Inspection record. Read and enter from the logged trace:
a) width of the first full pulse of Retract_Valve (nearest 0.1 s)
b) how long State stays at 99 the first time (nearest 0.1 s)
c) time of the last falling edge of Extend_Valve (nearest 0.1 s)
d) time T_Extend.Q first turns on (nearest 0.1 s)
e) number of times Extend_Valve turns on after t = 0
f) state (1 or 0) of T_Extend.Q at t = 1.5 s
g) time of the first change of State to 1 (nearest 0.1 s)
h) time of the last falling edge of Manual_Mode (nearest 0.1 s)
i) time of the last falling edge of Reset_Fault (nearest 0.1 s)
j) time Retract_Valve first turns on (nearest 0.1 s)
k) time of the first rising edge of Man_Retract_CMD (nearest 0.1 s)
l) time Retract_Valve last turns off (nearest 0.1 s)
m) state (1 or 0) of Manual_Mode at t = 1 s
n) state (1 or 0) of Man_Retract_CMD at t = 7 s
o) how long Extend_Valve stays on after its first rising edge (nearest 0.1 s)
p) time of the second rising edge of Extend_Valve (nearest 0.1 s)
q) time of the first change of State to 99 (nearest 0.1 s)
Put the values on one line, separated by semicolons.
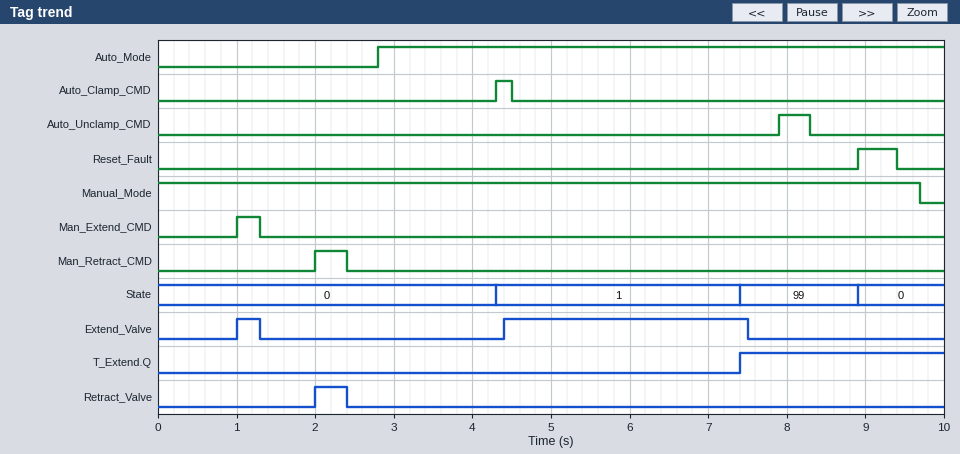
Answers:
0.4 s; 1.5 s; 7.5 s; 7.4 s; 2; 0; 4.3 s; 9.7 s; 9.4 s; 2.0 s; 2.0 s; 2.4 s; 1; 0; 0.3 s; 4.4 s; 7.4 s
